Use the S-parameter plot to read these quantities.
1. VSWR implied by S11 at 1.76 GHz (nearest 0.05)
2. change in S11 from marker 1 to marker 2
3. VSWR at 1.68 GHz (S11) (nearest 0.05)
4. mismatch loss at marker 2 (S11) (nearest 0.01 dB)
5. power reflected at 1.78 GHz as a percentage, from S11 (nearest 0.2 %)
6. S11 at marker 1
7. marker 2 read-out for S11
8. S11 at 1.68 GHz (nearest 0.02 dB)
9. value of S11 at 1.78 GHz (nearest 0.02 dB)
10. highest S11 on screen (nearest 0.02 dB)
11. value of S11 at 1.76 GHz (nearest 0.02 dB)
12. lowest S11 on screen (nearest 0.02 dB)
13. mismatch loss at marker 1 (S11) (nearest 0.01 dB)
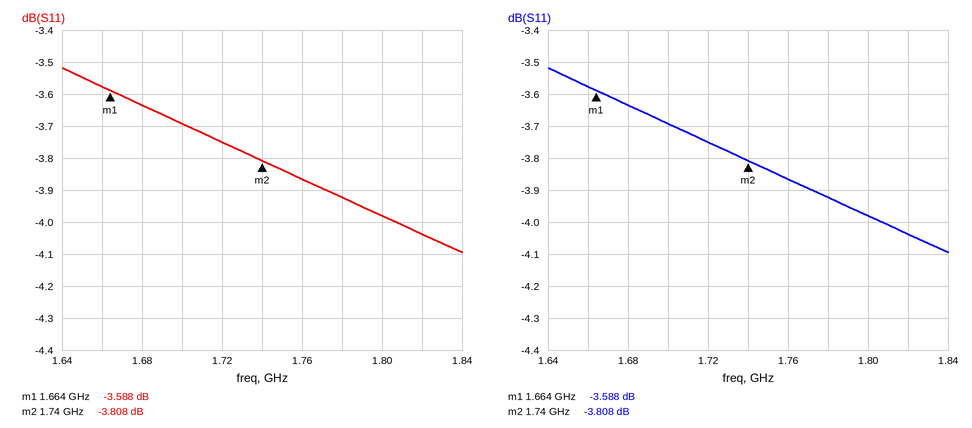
4.55
-0.220 dB
4.85
2.34 dB
40.6 %
-3.588 dB
-3.808 dB
-3.64 dB
-3.92 dB
-3.52 dB
-3.86 dB
-4.10 dB
2.50 dB
